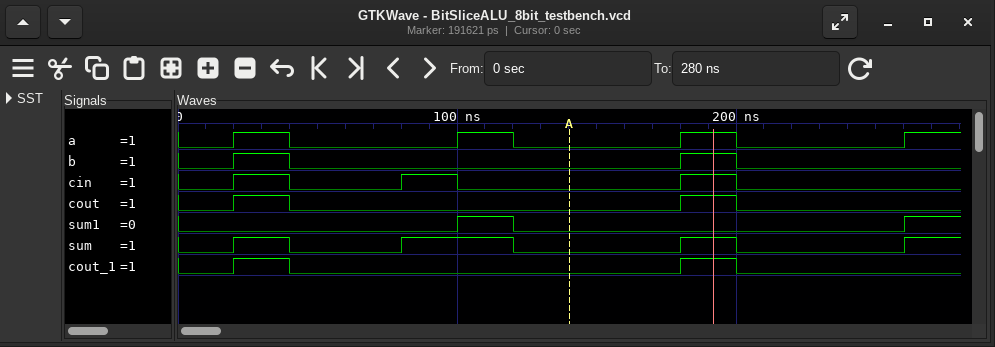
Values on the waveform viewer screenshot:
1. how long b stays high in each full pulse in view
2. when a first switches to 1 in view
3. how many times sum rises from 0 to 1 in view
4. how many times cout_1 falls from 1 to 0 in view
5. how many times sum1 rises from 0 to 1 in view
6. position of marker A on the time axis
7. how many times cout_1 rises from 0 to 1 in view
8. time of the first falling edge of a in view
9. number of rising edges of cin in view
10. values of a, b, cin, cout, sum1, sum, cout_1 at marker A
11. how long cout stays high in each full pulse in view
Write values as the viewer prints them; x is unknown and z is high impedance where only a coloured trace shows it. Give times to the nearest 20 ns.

20 ns, 20 ns
20 ns
4
2
2
140 ns
2
40 ns
3
a=0, b=0, cin=0, cout=0, sum1=0, sum=0, cout_1=0
20 ns, 20 ns
